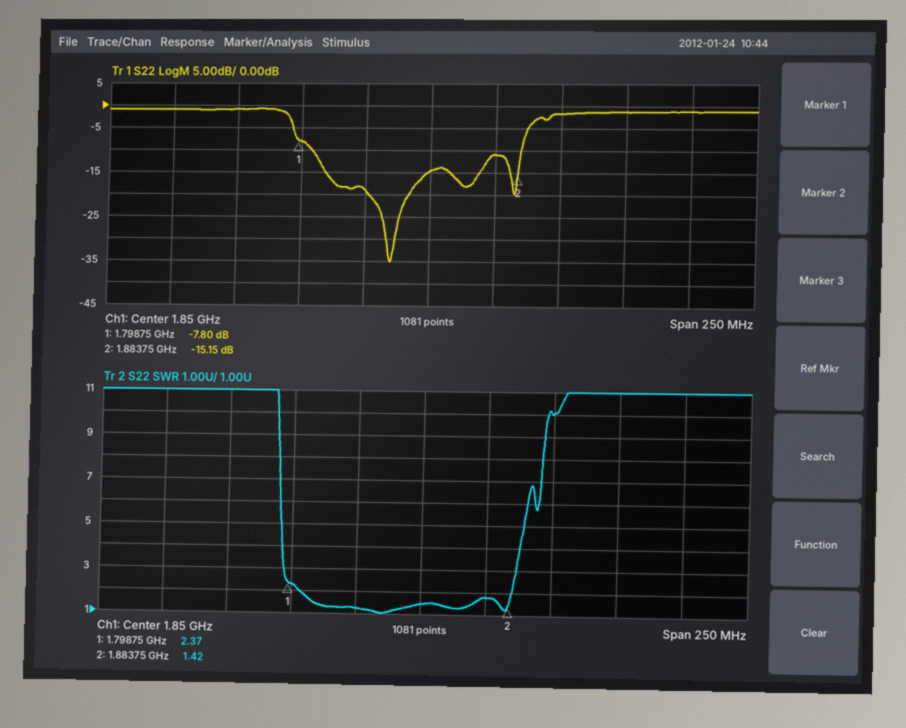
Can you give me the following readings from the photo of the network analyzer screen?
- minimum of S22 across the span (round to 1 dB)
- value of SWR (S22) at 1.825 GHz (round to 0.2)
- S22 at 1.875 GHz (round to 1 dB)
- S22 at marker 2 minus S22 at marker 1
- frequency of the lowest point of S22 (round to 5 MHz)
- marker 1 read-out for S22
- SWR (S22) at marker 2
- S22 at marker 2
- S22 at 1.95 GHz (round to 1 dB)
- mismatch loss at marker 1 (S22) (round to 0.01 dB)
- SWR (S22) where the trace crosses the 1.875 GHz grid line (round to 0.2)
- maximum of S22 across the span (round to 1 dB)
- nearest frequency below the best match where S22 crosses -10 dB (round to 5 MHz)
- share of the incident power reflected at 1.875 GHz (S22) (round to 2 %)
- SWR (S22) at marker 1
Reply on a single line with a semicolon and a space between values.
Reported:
-35 dB; 1.2; -11 dB; -7.35 dB; 1.835 GHz; -7.80 dB; 1.42; -15.15 dB; -1 dB; 0.79 dB; 1.8; -1 dB; 1.805 GHz; 8 %; 2.37
